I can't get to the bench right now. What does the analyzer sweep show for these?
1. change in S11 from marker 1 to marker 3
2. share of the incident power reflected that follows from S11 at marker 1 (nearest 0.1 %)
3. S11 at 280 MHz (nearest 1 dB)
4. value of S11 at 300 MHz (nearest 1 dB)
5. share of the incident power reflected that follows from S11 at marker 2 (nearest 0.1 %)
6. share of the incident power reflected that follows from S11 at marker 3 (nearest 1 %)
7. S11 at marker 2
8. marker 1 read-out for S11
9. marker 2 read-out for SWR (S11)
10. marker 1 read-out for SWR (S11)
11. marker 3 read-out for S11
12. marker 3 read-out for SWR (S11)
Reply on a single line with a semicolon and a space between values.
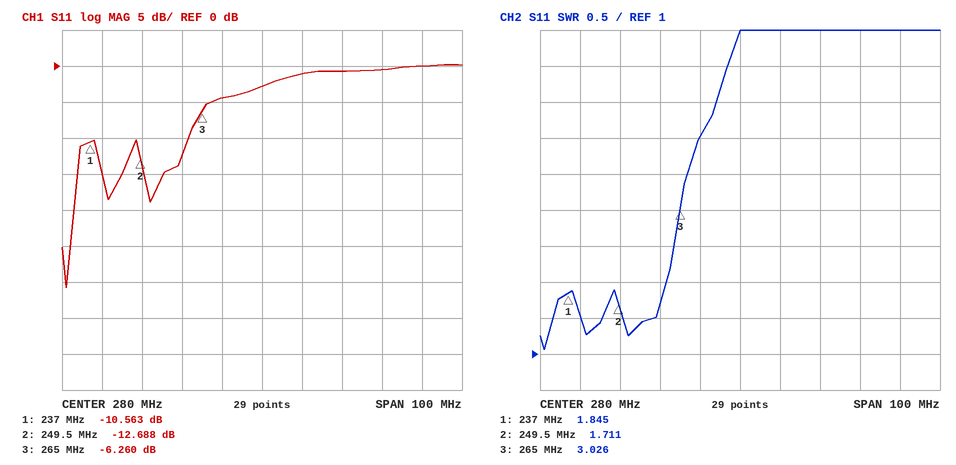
4.303 dB; 8.8 %; -3 dB; -1 dB; 5.4 %; 24 %; -12.688 dB; -10.563 dB; 1.711; 1.845; -6.260 dB; 3.026
